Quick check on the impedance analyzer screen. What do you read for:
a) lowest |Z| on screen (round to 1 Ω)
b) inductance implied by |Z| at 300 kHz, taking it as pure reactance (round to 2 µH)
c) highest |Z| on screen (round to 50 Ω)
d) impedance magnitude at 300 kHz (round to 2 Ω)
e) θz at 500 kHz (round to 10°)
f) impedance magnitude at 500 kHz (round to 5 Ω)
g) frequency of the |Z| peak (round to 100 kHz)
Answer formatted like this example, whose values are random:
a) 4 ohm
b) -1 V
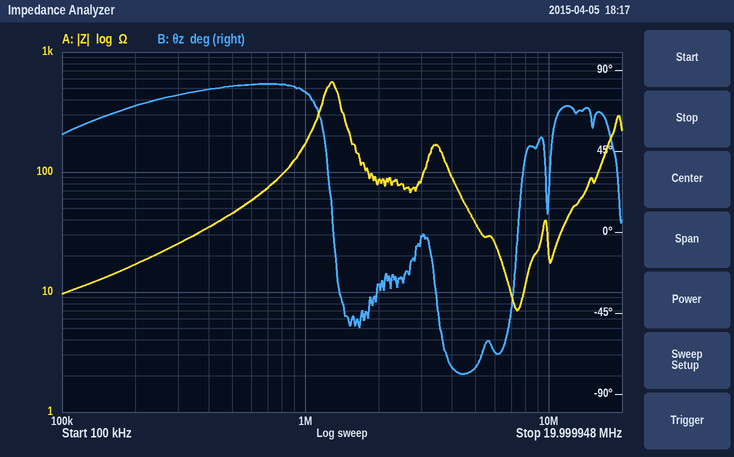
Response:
a) 7 Ω
b) 14 µH
c) 550 Ω
d) 26 Ω
e) 80°
f) 45 Ω
g) 1.3 MHz
